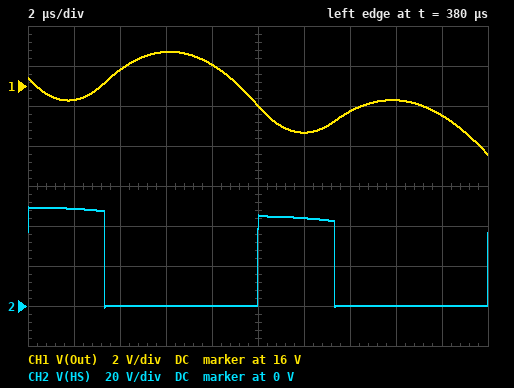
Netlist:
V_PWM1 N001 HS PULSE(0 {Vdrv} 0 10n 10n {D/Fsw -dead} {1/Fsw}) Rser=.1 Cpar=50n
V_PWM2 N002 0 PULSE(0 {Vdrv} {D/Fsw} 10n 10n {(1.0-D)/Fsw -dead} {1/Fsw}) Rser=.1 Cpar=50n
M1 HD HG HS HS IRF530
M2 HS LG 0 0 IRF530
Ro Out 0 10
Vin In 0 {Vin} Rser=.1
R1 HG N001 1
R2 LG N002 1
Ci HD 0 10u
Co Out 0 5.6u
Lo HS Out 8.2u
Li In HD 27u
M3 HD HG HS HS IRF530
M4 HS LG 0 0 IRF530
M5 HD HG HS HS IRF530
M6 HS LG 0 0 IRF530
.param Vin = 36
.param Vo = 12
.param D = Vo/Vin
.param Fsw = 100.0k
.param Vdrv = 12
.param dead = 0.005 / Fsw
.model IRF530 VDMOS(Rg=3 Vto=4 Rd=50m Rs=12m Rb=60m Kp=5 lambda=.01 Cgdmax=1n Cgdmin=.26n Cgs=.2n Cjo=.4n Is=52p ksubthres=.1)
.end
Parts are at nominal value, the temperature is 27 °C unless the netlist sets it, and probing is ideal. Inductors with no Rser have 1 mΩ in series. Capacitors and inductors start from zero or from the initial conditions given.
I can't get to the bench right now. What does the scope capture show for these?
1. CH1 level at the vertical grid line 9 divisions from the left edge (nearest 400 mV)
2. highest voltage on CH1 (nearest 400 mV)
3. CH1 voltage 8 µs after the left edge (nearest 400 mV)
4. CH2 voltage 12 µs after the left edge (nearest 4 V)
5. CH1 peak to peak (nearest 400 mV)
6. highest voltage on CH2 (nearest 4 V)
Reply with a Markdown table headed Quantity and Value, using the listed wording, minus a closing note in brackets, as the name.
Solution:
| Quantity | Value |
|---|---|
| CH1 level at the vertical grid line 9 divisions from the left edge | 14.4 V |
| highest voltage on CH1 | 17.6 V |
| CH1 voltage 8 µs after the left edge | 17.2 V |
| CH2 voltage 12 µs after the left edge | 44 V |
| CH1 peak to peak | 5.2 V |
| highest voltage on CH2 | 48 V |
